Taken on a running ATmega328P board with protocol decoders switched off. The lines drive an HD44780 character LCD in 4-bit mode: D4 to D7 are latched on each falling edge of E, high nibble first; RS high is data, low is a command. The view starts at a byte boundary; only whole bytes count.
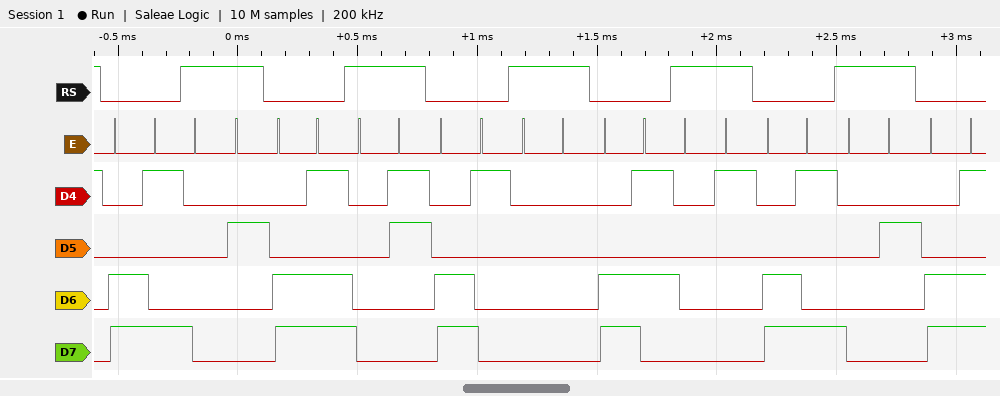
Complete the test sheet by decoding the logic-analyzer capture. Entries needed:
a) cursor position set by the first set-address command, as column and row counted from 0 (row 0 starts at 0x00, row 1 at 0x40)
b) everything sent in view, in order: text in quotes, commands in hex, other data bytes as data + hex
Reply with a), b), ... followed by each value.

a) column 9, row 1
b) 0xC9 data 02 0xCD data 03 0xC1 data 00 0xC5 data 01 0xC9 data 02 0xCD
